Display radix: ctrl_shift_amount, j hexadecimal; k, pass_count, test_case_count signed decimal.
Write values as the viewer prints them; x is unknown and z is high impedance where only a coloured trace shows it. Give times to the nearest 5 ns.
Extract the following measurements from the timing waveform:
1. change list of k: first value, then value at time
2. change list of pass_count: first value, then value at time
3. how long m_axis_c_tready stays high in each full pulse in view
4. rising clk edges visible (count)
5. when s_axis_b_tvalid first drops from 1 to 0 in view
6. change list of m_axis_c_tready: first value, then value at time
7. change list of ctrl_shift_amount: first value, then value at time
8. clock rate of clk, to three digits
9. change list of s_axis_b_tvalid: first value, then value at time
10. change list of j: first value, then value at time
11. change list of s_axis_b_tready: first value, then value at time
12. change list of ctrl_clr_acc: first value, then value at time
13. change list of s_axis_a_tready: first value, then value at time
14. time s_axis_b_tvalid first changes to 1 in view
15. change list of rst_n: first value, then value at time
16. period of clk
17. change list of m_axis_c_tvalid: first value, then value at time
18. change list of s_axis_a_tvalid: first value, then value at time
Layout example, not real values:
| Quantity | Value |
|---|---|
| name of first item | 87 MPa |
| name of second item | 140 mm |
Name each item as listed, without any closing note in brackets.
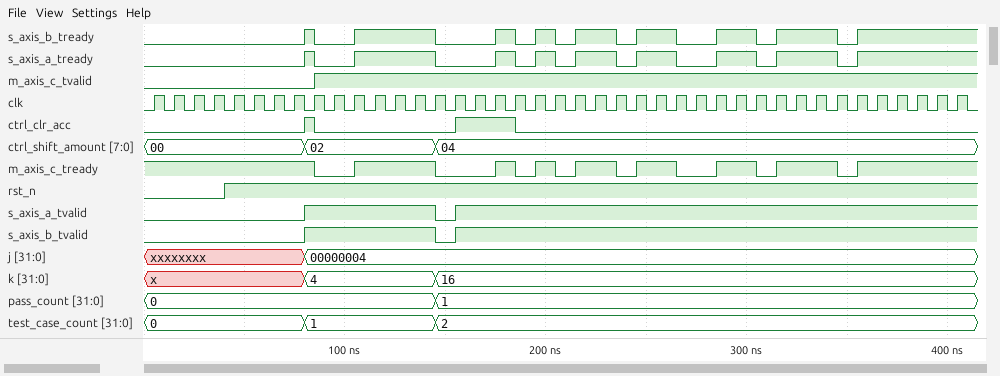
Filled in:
| Quantity | Value |
|---|---|
| change list of k: first value, then value at time | x, 4 at 80 ns, 16 at 145 ns |
| change list of pass_count: first value, then value at time | 0, 1 at 145 ns |
| how long m_axis_c_tready stays high in each full pulse in view | 40 ns, 10 ns, 10 ns, 20 ns, 20 ns, 20 ns, 30 ns |
| rising clk edges visible | 41 |
| when s_axis_b_tvalid first drops from 1 to 0 in view | 145 ns |
| change list of m_axis_c_tready: first value, then value at time | 1, 0 at 85 ns, 1 at 105 ns, 0 at 145 ns, 1 at 175 ns, 0 at 185 ns, 1 at 195 ns, 0 at 205 ns, 1 at 215 ns, 0 at 235 ns, 1 at 245 ns, 0 at 265 ns, 1 at 285 ns, 0 at 305 ns, 1 at 315 ns, 0 at 345 ns, 1 at 355 ns |
| change list of ctrl_shift_amount: first value, then value at time | 00, 02 at 80 ns, 04 at 145 ns |
| clock rate of clk, to three digits | 100 MHz |
| change list of s_axis_b_tvalid: first value, then value at time | 0, 1 at 80 ns, 0 at 145 ns, 1 at 155 ns |
| change list of j: first value, then value at time | xxxxxxxx, 00000004 at 80 ns |
| change list of s_axis_b_tready: first value, then value at time | 0, 1 at 80 ns, 0 at 85 ns, 1 at 105 ns, 0 at 145 ns, 1 at 175 ns, 0 at 185 ns, 1 at 195 ns, 0 at 205 ns, 1 at 215 ns, 0 at 235 ns, 1 at 245 ns, 0 at 265 ns, 1 at 285 ns, 0 at 305 ns, 1 at 315 ns, 0 at 345 ns, 1 at 355 ns |
| change list of ctrl_clr_acc: first value, then value at time | 0, 1 at 80 ns, 0 at 85 ns, 1 at 155 ns, 0 at 185 ns |
| change list of s_axis_a_tready: first value, then value at time | 0, 1 at 80 ns, 0 at 85 ns, 1 at 105 ns, 0 at 145 ns, 1 at 175 ns, 0 at 185 ns, 1 at 195 ns, 0 at 205 ns, 1 at 215 ns, 0 at 235 ns, 1 at 245 ns, 0 at 265 ns, 1 at 285 ns, 0 at 305 ns, 1 at 315 ns, 0 at 345 ns, 1 at 355 ns |
| time s_axis_b_tvalid first changes to 1 in view | 80 ns |
| change list of rst_n: first value, then value at time | 0, 1 at 40 ns |
| period of clk | 10 ns |
| change list of m_axis_c_tvalid: first value, then value at time | 0, 1 at 85 ns |
| change list of s_axis_a_tvalid: first value, then value at time | 0, 1 at 80 ns, 0 at 145 ns, 1 at 155 ns |
